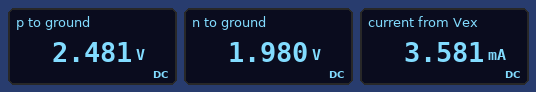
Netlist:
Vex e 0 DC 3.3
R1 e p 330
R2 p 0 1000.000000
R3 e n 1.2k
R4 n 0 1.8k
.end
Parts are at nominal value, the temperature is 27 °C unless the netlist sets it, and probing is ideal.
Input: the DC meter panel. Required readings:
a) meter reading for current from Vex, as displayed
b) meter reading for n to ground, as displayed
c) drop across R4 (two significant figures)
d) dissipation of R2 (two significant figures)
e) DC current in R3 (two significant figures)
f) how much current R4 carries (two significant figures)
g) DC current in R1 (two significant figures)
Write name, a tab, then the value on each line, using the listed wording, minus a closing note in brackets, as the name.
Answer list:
meter reading for current from Vex, as displayed	3.581 mA
meter reading for n to ground, as displayed	1.980 V
drop across R4	2.0 V
dissipation of R2	6.2 mW
DC current in R3	1.1 mA
how much current R4 carries	1.1 mA
DC current in R1	2.5 mA
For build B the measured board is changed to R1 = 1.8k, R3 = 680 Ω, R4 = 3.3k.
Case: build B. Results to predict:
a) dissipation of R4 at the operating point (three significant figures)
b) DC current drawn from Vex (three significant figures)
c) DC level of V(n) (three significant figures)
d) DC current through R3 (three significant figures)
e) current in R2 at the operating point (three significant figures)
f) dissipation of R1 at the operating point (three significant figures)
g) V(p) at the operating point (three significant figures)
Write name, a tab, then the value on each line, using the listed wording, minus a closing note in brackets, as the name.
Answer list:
dissipation of R4 at the operating point	2.27 mW
DC current drawn from Vex	2.01 mA
DC level of V(n)	2.74 V
DC current through R3	829 µA
current in R2 at the operating point	1.18 mA
dissipation of R1 at the operating point	2.50 mW
V(p) at the operating point	1.18 V
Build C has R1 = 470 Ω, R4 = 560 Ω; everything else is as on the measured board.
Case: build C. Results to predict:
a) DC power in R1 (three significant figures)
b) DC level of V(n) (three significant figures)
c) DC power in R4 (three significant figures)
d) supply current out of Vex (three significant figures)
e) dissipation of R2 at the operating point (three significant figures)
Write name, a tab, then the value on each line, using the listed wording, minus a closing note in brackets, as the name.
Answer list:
DC power in R1	2.37 mW
DC level of V(n)	1.05 V
DC power in R4	1.97 mW
supply current out of Vex	4.12 mA
dissipation of R2 at the operating point	5.04 mW
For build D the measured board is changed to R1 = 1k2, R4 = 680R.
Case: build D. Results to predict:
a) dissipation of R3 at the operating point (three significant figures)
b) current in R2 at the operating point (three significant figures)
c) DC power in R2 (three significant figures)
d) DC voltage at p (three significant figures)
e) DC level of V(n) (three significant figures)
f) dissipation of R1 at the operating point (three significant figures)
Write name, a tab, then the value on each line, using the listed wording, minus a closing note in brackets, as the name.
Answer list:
dissipation of R3 at the operating point	3.70 mW
current in R2 at the operating point	1.50 mA
DC power in R2	2.25 mW
DC voltage at p	1.50 V
DC level of V(n)	1.19 V
dissipation of R1 at the operating point	2.70 mW
